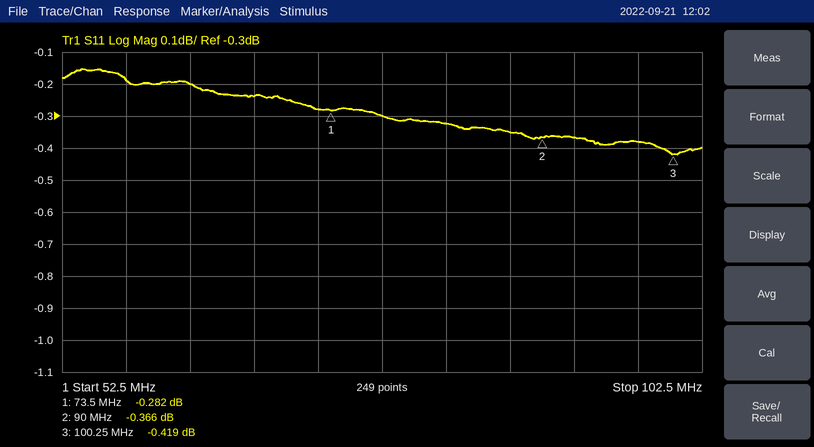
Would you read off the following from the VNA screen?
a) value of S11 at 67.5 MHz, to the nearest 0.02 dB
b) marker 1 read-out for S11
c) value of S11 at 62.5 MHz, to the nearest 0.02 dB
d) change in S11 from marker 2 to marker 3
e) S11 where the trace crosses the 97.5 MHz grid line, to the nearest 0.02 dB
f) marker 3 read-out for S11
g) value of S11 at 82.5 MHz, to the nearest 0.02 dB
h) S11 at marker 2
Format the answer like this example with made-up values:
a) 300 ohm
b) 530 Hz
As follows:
a) -0.24 dB
b) -0.282 dB
c) -0.20 dB
d) -0.053 dB
e) -0.38 dB
f) -0.419 dB
g) -0.32 dB
h) -0.366 dB
